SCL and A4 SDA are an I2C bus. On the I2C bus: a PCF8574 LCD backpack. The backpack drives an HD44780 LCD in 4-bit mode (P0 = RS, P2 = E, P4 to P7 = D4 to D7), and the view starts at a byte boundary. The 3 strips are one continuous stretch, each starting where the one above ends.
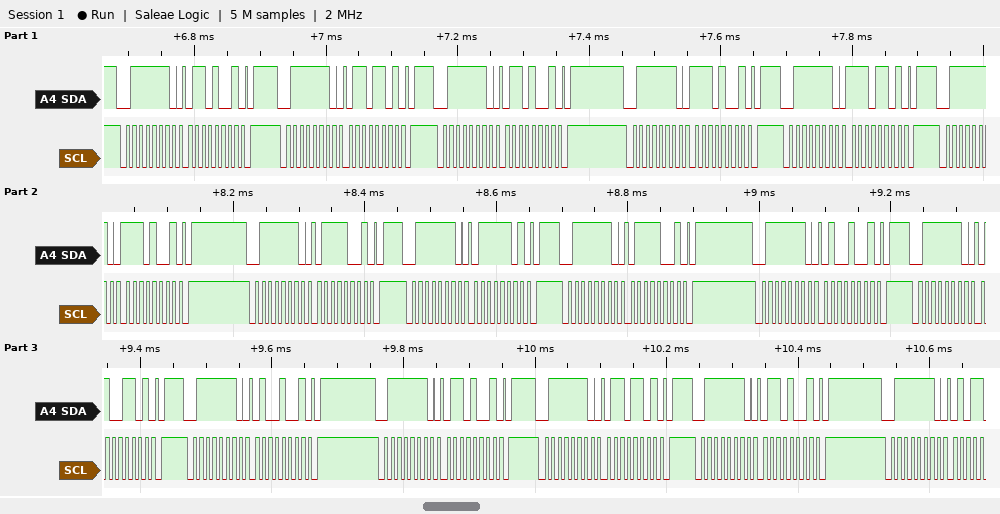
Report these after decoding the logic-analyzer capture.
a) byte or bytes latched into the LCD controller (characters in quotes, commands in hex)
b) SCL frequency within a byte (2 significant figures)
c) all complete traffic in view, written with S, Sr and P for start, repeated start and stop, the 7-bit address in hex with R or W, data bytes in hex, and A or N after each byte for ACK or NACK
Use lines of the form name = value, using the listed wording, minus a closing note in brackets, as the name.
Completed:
byte or bytes latched into the LCD controller = 'n' 't'
SCL frequency within a byte = 100 kHz
all complete traffic in view, written with S, Sr and P for start, repeated start and stop, the 7-bit address in hex with R or W, data bytes in hex, and A or N after each byte for ACK or NACK = S 3FW A 69 A P S 3FW A 6D A P S 3FW A 69 A P S 3FW A E9 A P S 3FW A ED A P S 3FW A E9 A P S 3FW A 79 A P S 3FW A 7D A P S 3FW A 79 A P S 3FW A 49 A P S 3FW A 4D A P S 3FW A 49 A P S 3FW A 69 A P S 3FW A 6D A P S 3FW A 69 A P S 3FW A
